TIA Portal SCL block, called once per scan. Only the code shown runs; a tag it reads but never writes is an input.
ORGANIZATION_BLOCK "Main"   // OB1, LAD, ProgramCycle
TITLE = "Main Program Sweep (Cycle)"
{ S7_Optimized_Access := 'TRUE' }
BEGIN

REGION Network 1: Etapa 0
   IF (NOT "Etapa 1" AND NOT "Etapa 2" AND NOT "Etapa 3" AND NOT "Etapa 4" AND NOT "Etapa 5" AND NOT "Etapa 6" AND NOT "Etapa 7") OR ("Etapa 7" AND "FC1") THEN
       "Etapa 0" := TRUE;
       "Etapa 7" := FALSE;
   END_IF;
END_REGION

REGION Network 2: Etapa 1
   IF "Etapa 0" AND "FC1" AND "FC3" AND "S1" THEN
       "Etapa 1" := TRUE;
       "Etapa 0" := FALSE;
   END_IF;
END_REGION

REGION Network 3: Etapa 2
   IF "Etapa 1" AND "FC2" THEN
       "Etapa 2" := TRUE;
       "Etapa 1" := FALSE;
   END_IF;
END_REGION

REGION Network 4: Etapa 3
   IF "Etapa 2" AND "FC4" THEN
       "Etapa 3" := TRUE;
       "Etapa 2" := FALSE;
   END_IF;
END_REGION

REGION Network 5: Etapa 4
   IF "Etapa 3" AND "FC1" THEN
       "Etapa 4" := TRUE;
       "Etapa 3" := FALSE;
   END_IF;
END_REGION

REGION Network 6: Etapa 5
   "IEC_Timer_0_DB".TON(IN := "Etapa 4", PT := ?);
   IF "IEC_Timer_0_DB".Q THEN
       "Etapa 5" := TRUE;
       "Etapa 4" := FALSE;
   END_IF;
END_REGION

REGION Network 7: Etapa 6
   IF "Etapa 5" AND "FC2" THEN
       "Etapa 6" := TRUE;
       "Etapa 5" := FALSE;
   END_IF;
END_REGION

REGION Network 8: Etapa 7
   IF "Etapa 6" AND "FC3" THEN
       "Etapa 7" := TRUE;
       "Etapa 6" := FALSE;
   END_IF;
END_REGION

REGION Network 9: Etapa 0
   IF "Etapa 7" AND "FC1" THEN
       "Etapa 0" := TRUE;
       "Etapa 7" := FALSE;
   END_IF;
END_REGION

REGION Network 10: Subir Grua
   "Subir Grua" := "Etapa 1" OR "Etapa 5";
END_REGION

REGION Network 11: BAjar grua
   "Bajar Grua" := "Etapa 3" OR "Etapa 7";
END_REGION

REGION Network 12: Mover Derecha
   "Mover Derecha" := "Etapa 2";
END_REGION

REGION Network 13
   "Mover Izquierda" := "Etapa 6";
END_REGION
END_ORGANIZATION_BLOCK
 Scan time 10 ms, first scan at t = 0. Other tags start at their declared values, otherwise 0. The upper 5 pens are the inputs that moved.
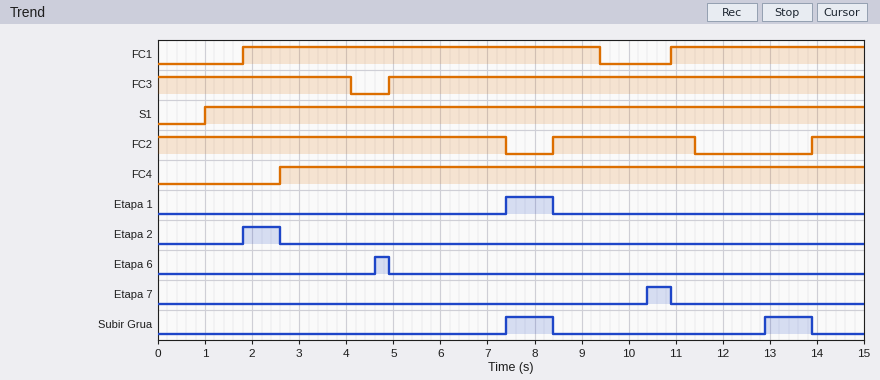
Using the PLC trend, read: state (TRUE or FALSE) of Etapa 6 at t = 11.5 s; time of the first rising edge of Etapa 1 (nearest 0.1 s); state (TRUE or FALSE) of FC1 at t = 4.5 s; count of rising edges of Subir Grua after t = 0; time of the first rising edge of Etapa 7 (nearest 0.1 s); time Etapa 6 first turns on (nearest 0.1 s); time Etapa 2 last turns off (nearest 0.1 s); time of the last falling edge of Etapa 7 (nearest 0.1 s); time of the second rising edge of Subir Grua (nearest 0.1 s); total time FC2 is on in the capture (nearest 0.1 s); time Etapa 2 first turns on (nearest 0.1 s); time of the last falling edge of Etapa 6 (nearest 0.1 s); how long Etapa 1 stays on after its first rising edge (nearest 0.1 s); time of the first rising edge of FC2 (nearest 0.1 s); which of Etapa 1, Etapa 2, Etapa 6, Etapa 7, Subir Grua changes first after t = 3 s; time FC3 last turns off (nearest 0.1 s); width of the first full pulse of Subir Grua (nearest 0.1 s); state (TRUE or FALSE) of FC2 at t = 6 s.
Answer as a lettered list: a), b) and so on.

a) FALSE
b) 7.4 s
c) TRUE
d) 2
e) 10.4 s
f) 4.6 s
g) 2.6 s
h) 10.9 s
i) 12.9 s
j) 11.5 s
k) 1.8 s
l) 4.9 s
m) 1.0 s
n) 8.4 s
o) Etapa 6
p) 4.1 s
q) 1.0 s
r) TRUE
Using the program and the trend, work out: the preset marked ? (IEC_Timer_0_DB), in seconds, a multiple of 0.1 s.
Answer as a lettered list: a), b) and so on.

a) 2.0 s
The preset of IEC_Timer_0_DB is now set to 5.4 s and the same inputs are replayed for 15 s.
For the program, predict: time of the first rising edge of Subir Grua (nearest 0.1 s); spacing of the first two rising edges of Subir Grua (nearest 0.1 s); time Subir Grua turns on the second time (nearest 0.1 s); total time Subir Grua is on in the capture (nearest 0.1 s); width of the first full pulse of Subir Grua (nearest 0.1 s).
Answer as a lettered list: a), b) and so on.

a) 8.0 s
b) 5.8 s
c) 13.8 s
d) 0.5 s
e) 0.4 s
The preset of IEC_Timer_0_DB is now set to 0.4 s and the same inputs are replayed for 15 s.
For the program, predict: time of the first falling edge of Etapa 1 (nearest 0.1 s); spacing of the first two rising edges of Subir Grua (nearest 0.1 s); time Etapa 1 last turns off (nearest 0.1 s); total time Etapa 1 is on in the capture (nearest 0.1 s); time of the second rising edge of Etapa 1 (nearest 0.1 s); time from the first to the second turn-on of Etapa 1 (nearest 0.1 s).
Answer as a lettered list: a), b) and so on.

a) 8.4 s
b) 4.0 s
c) 13.9 s
d) 3.5 s
e) 11.4 s
f) 4.0 s
